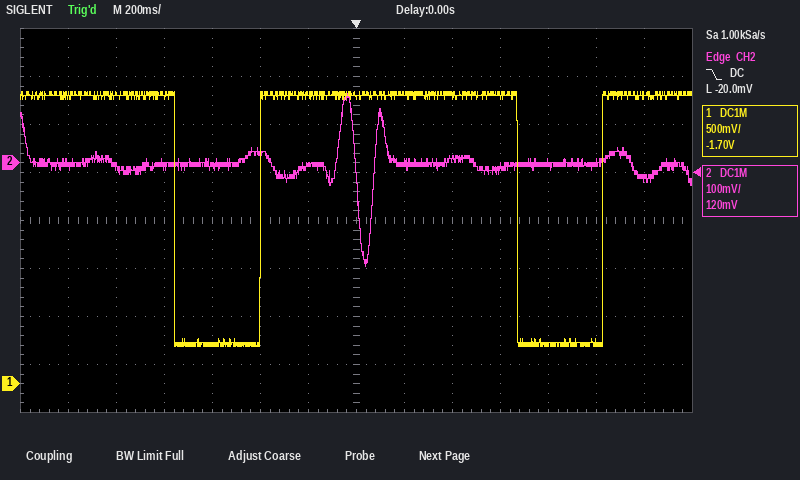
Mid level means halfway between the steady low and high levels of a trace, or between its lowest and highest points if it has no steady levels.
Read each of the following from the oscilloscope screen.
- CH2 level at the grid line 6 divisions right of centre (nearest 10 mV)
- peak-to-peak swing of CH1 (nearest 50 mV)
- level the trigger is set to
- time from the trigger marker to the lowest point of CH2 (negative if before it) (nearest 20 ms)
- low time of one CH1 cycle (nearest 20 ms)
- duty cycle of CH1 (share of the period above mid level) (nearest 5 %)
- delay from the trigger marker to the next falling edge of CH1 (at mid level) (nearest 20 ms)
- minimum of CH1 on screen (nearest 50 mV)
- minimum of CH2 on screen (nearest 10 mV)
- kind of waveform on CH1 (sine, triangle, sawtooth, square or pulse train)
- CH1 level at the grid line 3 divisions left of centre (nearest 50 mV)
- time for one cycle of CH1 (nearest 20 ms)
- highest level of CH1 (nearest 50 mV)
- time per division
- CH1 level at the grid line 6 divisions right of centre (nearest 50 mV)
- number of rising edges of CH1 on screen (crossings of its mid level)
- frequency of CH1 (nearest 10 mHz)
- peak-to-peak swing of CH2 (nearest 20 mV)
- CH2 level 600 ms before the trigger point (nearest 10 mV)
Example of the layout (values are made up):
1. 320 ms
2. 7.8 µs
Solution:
1. -30 mV
2. 2.65 V
3. -20.0 mV
4. +40 ms
5. 360 ms
6. 75 %
7. 680 ms
8. 400 mV
9. -220 mV
10. pulse train
11. 400 mV
12. 1.42 s
13. 3.05 V
14. 200 ms
15. 3.00 V
16. 2
17. 700 mHz
18. 360 mV
19. -10 mV
